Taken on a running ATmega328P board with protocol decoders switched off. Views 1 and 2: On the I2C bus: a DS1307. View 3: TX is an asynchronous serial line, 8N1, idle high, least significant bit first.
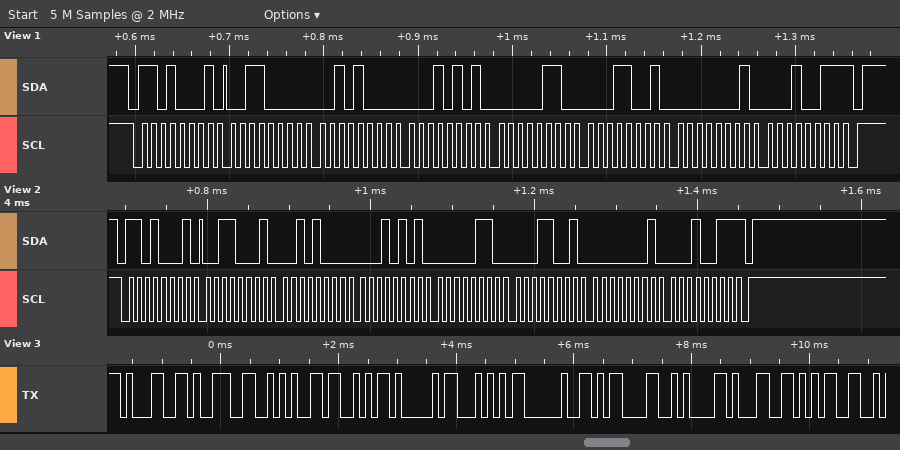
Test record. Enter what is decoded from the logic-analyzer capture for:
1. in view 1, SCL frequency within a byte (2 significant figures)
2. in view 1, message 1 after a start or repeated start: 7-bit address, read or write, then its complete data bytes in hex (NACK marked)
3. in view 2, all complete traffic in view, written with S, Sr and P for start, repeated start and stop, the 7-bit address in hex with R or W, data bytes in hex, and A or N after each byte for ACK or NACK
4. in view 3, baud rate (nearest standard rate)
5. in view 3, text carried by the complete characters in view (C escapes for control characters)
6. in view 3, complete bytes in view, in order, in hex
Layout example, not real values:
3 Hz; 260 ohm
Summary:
100 kHz; 0x68 read: 30 28 15 06 19 01 13 NACK; S 68R A 31 A 28 A 15 A 06 A 19 A 01 A 13 N P; 9600 baud; "19*SAT \r\n15"; 31 39 2A 53 41 54 20 0D 0A 31 35
